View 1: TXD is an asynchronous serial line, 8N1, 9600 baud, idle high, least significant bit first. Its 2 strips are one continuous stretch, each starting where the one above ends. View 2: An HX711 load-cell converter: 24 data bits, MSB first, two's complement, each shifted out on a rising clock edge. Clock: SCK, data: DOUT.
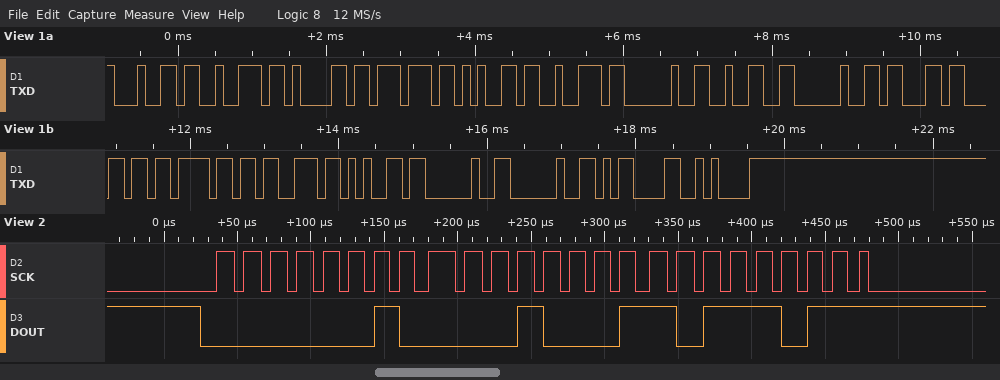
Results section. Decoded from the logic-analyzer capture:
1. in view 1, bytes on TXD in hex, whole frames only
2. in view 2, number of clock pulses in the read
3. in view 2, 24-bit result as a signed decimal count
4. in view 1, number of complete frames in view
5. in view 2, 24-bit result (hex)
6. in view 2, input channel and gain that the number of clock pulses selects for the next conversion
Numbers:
64 72 61 77 65 72 20 32 20 63 6C 6F 73 65 20 20 0D 0A
25
135611
18
0x0211BB
channel A, gain 128
